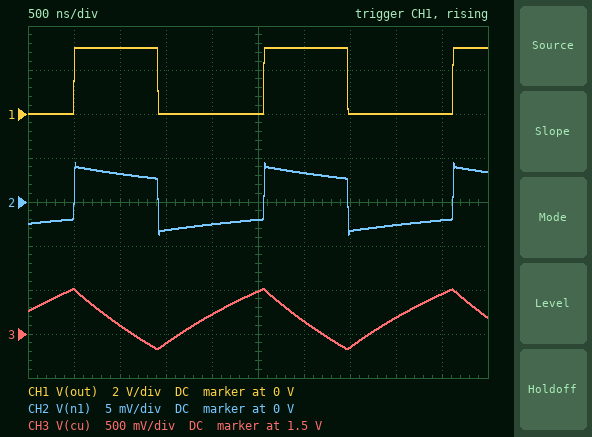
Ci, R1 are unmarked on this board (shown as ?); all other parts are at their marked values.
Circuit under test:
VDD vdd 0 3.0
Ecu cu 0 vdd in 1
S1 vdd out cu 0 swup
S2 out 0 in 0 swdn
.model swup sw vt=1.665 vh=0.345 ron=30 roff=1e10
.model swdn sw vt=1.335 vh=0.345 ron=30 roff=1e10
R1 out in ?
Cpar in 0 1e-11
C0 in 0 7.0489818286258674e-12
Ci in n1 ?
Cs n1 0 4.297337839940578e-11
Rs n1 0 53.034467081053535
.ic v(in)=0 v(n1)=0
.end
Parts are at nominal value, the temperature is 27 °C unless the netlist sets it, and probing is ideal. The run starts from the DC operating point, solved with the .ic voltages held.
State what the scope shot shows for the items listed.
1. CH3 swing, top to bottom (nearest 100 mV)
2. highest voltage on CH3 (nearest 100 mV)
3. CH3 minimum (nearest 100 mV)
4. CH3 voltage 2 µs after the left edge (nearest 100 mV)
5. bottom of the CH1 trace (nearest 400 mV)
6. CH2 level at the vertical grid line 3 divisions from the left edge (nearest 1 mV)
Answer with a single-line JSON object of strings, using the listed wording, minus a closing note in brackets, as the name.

{"CH3 swing, top to bottom": "700 mV", "highest voltage on CH3": "2.0 V", "CH3 minimum": "1.3 V", "CH3 voltage 2 µs after the left edge": "1.7 V", "bottom of the CH1 trace": "0 V", "CH2 level at the vertical grid line 3 divisions from the left edge": "-3 mV"}
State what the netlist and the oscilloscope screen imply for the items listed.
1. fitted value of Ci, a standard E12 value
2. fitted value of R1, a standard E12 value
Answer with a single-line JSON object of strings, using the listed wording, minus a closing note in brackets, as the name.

{"fitted value of Ci, a standard E12 value": "82 pF", "fitted value of R1, a standard E12 value": "22 kΩ"}
